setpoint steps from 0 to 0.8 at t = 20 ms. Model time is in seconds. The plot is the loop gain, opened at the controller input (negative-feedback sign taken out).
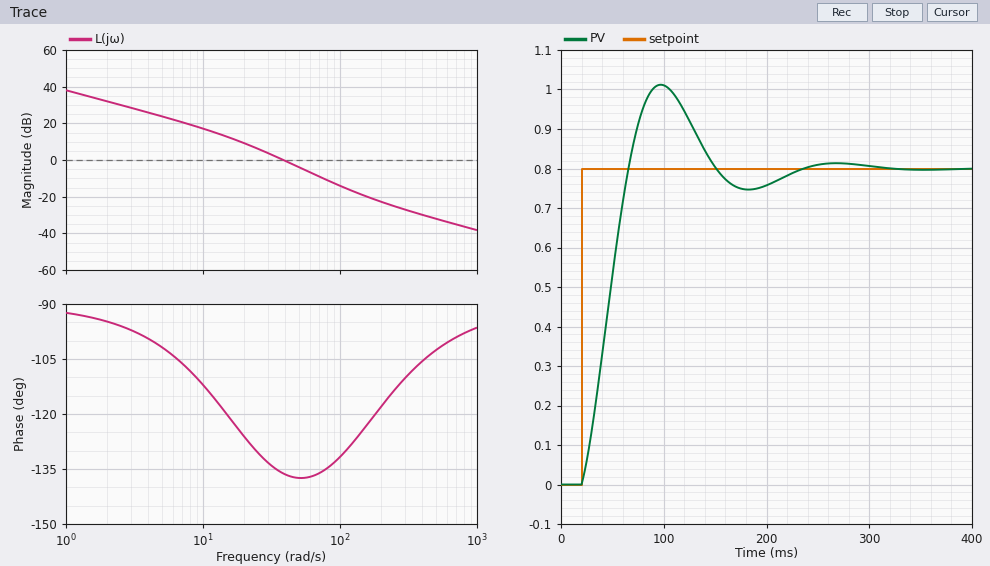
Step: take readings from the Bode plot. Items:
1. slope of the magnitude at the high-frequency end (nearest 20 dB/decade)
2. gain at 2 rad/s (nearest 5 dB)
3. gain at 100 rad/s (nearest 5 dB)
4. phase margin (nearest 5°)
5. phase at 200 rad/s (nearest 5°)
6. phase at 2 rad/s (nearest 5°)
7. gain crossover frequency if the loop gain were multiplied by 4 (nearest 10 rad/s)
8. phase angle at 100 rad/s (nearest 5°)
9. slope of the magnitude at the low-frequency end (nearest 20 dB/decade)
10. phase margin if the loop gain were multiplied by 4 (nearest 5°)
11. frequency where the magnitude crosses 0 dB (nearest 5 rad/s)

-20 dB/decade
30 dB
-15 dB
45°
-120°
-95°
90 rad/s
-130°
-20 dB/decade
45°
40 rad/s
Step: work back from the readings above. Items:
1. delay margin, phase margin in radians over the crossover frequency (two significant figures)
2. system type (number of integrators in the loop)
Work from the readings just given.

0.020 s
1
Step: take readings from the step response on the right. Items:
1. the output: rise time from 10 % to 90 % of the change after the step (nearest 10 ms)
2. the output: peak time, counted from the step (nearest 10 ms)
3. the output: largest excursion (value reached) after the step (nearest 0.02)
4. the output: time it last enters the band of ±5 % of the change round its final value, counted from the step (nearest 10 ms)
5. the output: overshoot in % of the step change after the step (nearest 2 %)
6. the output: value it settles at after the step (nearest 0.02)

30 ms
80 ms
1.02
180 ms
26 %
0.80
